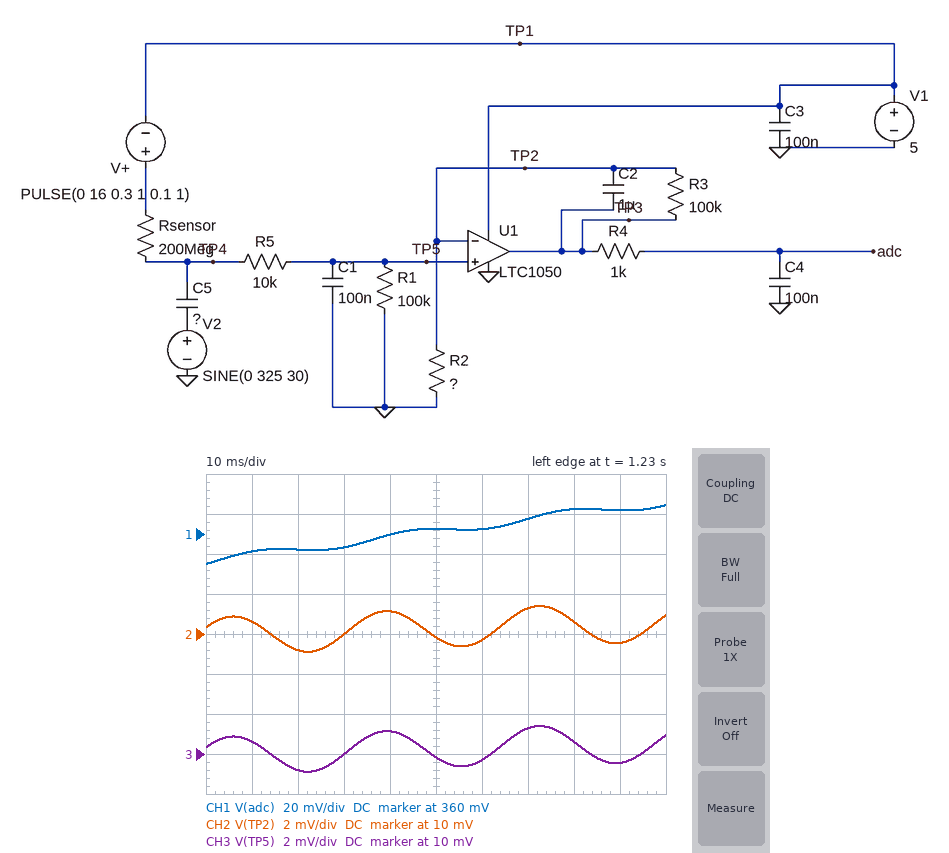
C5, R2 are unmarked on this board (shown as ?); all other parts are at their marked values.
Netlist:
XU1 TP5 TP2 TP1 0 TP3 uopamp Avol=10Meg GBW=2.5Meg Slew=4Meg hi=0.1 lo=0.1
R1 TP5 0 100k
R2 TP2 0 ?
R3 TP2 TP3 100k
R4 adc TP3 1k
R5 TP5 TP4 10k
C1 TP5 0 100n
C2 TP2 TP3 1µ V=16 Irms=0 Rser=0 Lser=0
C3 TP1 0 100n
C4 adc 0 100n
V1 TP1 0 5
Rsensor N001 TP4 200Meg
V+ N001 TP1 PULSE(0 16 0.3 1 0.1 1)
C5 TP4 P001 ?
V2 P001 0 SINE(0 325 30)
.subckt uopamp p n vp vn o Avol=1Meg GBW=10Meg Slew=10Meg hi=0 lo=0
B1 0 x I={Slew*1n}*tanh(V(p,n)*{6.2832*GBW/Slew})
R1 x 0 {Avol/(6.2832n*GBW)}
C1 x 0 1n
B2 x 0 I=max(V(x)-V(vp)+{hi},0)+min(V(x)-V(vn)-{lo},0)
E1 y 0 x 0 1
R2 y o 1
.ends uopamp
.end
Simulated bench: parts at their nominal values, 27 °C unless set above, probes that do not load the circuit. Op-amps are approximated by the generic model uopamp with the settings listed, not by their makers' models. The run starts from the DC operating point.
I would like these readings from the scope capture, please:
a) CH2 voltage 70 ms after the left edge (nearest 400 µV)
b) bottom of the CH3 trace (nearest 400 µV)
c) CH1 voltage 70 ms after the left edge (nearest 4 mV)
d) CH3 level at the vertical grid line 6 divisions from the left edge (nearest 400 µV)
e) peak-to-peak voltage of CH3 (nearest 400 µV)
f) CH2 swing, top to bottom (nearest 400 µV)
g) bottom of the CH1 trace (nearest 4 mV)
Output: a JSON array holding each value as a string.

["11.2 mV", "9.2 mV", "368 mV", "9.6 mV", "2.4 mV", "2.4 mV", "344 mV"]
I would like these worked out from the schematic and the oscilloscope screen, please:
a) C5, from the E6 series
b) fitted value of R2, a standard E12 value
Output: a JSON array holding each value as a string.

["330 fF", "2.7 kΩ"]
